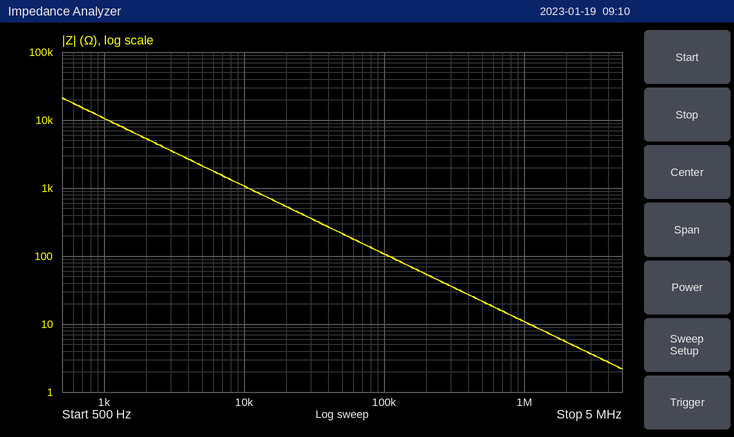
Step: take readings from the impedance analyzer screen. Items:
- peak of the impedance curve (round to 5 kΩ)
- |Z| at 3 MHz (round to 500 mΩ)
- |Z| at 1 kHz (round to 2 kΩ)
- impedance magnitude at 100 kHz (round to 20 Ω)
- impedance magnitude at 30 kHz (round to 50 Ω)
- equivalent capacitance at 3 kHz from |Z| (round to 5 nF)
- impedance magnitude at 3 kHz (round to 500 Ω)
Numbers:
20 kΩ
3.5 Ω
10 kΩ
100 Ω
350 Ω
15 nF
3.5 kΩ
